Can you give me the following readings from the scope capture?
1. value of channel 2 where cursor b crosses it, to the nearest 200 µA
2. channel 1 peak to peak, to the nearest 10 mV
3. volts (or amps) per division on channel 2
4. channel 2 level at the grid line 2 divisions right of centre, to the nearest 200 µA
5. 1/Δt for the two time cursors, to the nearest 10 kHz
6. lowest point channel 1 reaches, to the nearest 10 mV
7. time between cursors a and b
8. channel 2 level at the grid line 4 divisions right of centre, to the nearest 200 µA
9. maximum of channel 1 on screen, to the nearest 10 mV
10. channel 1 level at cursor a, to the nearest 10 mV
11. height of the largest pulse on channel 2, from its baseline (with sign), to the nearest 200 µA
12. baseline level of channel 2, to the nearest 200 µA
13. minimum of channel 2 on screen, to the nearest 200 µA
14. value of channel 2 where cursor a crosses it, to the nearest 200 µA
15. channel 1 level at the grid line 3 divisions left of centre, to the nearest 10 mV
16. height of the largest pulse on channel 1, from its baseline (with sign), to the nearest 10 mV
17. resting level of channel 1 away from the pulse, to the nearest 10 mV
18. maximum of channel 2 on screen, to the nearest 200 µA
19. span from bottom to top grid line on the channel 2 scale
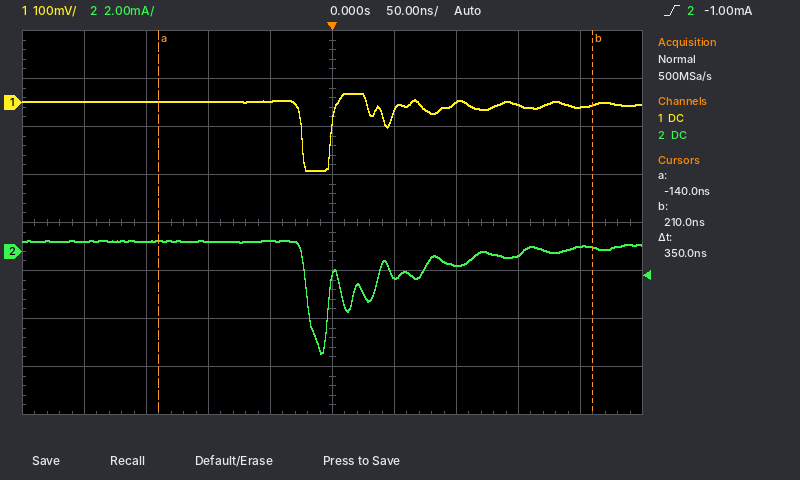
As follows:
200 µA
160 mV
2 mA
-600 µA
2.86 MHz
-140 mV
350 ns
200 µA
20 mV
0 mV
-4.6 mA
400 µA
-4.2 mA
400 µA
0 mV
-140 mV
0 mV
400 µA
16 mA
